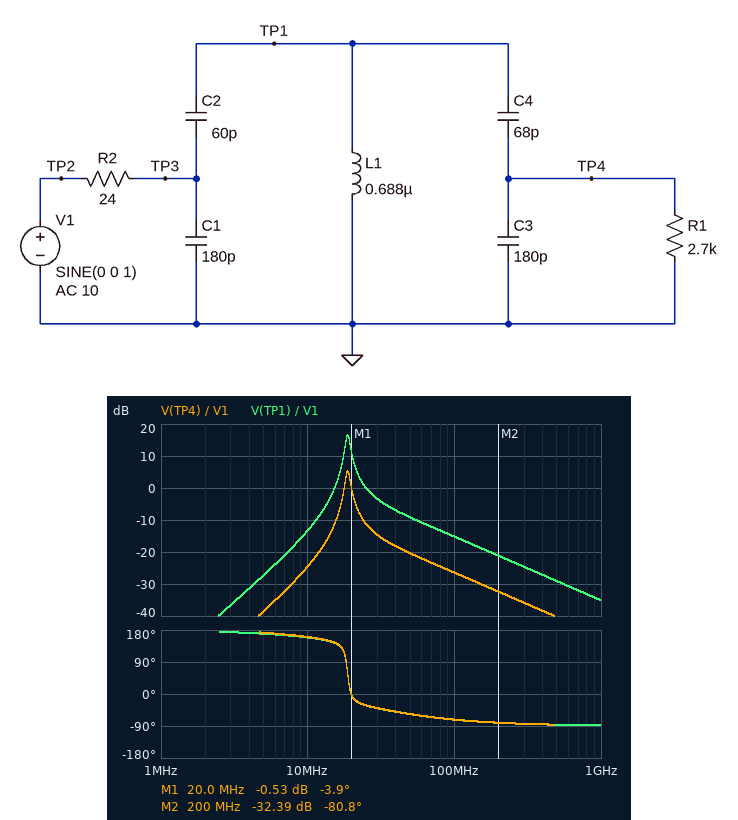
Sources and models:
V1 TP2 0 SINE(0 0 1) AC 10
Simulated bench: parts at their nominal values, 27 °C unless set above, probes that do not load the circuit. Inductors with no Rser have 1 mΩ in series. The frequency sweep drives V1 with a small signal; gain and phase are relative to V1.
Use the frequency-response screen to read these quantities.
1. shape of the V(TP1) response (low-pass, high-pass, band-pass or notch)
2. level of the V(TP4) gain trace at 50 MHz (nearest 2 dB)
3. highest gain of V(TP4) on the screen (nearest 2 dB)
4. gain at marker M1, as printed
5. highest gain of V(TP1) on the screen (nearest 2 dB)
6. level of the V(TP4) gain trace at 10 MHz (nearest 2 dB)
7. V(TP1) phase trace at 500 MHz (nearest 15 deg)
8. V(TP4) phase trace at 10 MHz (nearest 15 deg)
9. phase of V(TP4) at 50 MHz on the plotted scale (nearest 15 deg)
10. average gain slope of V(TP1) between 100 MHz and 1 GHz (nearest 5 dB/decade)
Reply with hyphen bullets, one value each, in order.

- band-pass
- -20 dB
- 6 dB
- -0.53 dB
- 16 dB
- -24 dB
- -90 deg
- 165 deg
- -60 deg
- -20 dB/decade
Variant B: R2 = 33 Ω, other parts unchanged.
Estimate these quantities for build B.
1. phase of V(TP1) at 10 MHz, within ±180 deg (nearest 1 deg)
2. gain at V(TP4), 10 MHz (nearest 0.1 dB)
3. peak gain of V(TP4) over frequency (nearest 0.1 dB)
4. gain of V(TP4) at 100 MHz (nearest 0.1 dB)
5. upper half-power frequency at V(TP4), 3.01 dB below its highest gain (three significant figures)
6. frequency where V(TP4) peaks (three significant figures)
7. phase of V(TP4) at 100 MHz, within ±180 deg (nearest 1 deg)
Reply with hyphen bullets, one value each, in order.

- 152 deg
- -25.0 dB
- 3.8 dB
- -29.0 dB
- 19.7 MHz
- 19.0 MHz
- -77 deg
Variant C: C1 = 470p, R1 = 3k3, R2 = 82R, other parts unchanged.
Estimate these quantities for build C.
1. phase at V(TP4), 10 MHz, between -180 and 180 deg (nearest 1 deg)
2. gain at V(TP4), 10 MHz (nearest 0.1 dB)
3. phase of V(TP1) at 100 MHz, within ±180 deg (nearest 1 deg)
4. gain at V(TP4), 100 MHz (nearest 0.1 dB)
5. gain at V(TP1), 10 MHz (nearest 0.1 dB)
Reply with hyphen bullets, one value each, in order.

- 111 deg
- -33.4 dB
- -88 deg
- -44.3 dB
- -22.2 dB
